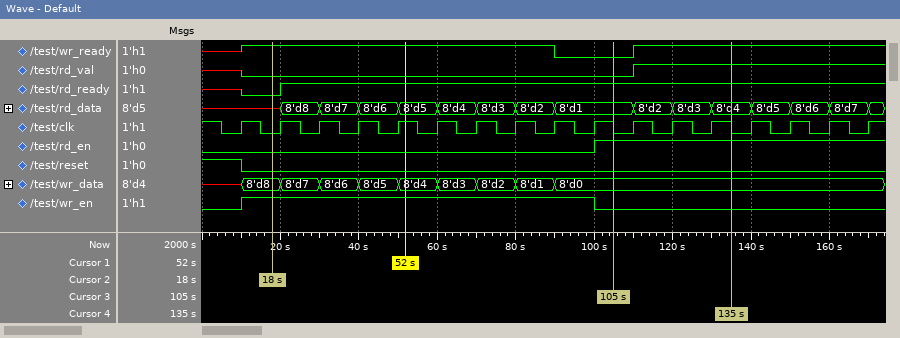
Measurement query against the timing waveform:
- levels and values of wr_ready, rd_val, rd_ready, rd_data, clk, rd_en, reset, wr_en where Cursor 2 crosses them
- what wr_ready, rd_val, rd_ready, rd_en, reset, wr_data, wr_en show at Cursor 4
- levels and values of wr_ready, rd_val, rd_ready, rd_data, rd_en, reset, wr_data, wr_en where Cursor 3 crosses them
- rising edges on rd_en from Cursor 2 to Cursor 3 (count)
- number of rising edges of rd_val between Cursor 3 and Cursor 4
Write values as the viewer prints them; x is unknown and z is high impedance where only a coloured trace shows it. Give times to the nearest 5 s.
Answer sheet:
wr_ready=1, rd_val=0, rd_ready=0, rd_data=x, clk=0, rd_en=0, reset=0, wr_en=1
wr_ready=1, rd_val=1, rd_ready=1, rd_en=1, reset=0, wr_data=8'd0, wr_en=0
wr_ready=0, rd_val=0, rd_ready=1, rd_data=8'd1, rd_en=1, reset=0, wr_data=8'd0, wr_en=0
1
1
